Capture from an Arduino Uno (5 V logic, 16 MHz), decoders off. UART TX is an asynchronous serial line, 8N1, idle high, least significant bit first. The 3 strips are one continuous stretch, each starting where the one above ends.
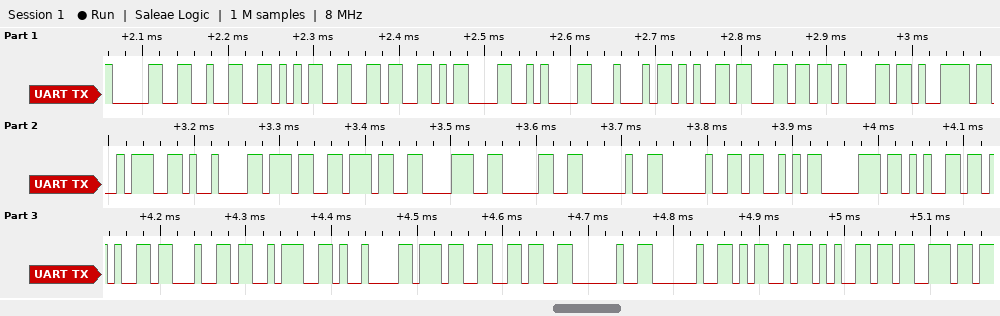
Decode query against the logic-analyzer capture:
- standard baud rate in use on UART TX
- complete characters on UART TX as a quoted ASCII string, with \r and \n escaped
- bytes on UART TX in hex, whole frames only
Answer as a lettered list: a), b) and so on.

a) 115200 baud
b) "0256\r\nDelay:\t7780  Speed:\t76  Mes"
c) 30 32 35 36 0D 0A 44 65 6C 61 79 3A 09 37 37 38 30 20 20 53 70 65 65 64 3A 09 37 36 20 20 4D 65 73
